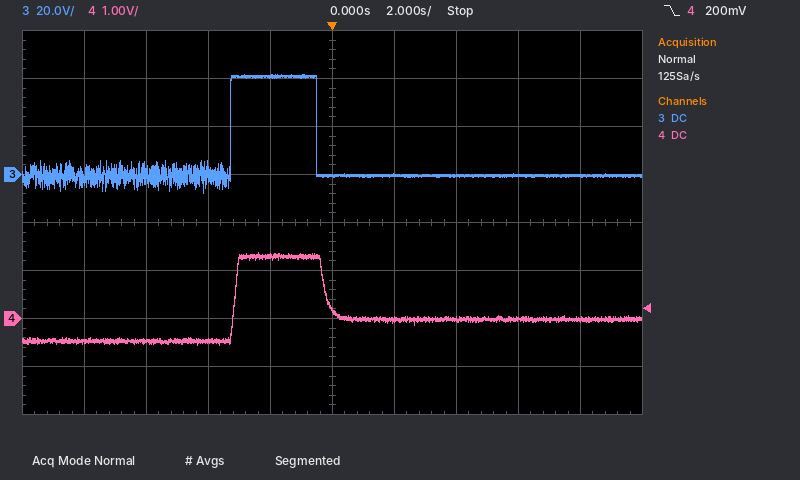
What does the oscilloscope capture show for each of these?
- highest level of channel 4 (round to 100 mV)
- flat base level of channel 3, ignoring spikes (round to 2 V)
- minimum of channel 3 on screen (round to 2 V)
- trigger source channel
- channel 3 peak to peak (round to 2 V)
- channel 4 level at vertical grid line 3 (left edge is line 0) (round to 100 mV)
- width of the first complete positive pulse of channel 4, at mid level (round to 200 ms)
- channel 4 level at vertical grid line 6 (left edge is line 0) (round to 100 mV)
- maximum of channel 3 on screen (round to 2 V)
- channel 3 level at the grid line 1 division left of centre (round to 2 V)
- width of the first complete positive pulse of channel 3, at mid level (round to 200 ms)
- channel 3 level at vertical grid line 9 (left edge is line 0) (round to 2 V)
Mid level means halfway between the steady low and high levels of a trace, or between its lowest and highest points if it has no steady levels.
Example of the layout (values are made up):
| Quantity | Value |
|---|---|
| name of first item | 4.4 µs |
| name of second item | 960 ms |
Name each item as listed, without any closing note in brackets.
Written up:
| Quantity | Value |
|---|---|
| highest level of channel 4 | 1.4 V |
| flat base level of channel 3, ignoring spikes | 0 V |
| minimum of channel 3 on screen | -8 V |
| trigger source channel | channel 4 |
| channel 3 peak to peak | 50 V |
| channel 4 level at vertical grid line 3 (left edge is line 0) | -500 mV |
| width of the first complete positive pulse of channel 4, at mid level | 3.0 s |
| channel 4 level at vertical grid line 6 (left edge is line 0) | 0.0 V |
| maximum of channel 3 on screen | 42 V |
| channel 3 level at the grid line 1 division left of centre | 42 V |
| width of the first complete positive pulse of channel 3, at mid level | 2.8 s |
| channel 3 level at vertical grid line 9 (left edge is line 0) | 0 V |
